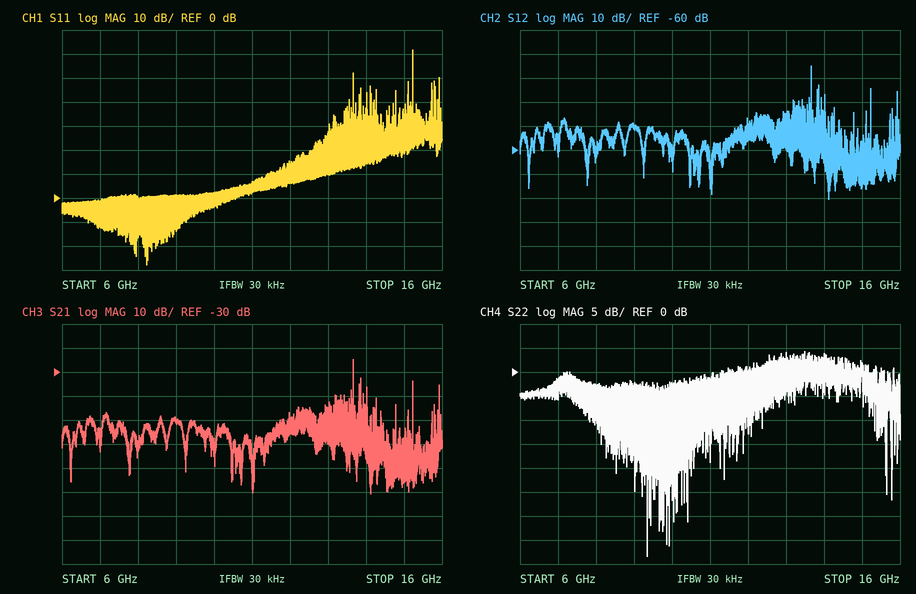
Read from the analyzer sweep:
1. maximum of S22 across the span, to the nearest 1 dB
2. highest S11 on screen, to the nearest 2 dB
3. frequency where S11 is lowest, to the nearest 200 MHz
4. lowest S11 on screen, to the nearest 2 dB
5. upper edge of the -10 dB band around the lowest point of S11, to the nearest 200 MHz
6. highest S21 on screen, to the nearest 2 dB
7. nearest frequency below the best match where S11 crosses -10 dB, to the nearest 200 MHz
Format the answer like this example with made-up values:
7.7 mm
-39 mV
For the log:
4 dB
62 dB
8.2 GHz
-28 dB
8.2 GHz
-24 dB
8.2 GHz
